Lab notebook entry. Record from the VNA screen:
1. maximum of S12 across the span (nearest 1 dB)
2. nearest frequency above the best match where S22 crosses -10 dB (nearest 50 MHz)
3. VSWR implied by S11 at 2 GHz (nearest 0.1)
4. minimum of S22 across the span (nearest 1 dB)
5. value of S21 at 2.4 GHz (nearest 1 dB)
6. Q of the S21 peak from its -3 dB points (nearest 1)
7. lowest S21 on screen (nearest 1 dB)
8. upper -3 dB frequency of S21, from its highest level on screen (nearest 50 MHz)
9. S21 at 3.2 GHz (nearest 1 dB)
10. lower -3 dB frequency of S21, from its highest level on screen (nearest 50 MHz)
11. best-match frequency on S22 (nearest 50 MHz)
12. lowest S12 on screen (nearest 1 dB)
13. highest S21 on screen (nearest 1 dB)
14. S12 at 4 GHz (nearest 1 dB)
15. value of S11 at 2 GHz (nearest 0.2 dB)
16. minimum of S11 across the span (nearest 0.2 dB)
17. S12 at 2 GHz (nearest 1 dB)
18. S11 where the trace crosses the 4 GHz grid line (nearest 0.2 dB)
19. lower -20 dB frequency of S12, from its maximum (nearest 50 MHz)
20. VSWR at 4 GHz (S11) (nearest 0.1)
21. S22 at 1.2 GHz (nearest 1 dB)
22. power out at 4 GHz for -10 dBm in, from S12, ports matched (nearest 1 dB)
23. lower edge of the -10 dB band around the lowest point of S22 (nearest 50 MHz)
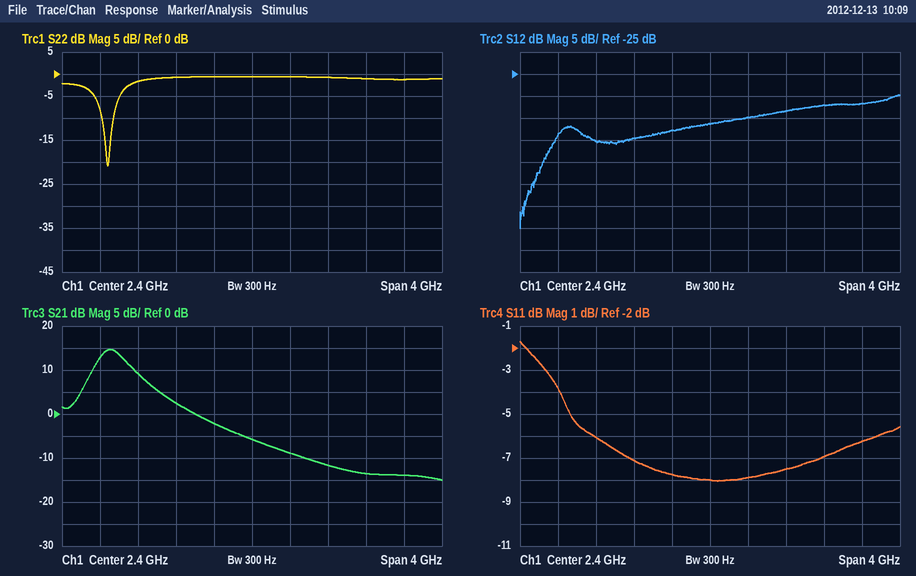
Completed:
-30 dB
950 MHz
2.4
-21 dB
-6 dB
3
-15 dB
1.10 GHz
-12 dB
750 MHz
900 MHz
-60 dB
15 dB
-32 dB
-7.8 dB
-8.0 dB
-38 dB
-6.2 dB
550 MHz
2.9
-2 dB
-42 dBm
800 MHz
